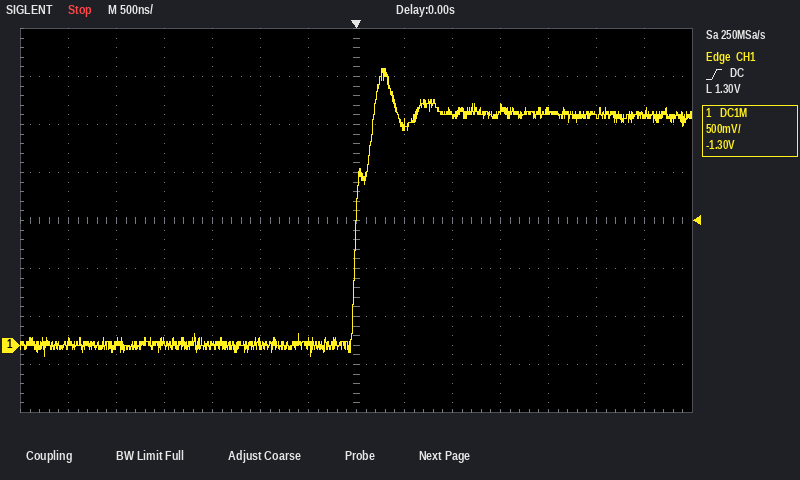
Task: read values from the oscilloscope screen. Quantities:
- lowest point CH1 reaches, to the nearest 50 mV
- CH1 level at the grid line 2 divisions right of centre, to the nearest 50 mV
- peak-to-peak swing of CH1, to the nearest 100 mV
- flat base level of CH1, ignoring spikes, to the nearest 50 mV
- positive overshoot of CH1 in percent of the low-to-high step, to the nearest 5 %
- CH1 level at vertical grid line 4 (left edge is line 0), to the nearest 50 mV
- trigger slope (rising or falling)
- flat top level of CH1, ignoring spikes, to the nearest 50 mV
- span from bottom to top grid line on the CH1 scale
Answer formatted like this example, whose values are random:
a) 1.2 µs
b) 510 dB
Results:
a) -100 mV
b) 2.40 V
c) 3.00 V
d) 0 mV
e) 20 %
f) 0 mV
g) rising
h) 2.40 V
i) 4 V
